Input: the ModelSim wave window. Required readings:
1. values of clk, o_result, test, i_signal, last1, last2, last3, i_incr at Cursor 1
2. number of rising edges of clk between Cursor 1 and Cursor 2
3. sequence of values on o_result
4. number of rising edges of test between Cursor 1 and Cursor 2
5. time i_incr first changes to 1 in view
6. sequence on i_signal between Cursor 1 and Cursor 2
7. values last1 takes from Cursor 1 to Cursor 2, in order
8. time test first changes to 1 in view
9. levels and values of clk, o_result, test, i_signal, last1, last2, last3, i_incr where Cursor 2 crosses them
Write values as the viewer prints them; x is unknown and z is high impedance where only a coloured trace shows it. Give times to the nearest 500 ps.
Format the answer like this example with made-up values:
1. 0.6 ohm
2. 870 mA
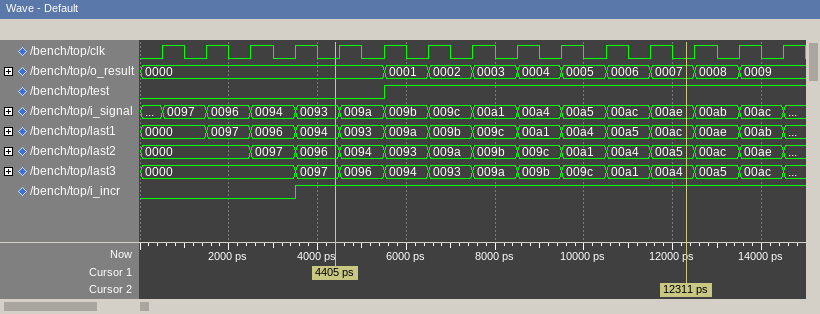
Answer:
1. clk=0, o_result=0000, test=0, i_signal=0093, last1=0094, last2=0096, last3=0097, i_incr=1
2. 8
3. 0000, 0001, 0002, 0003, 0004, 0005, 0006, 0007, 0008, 0009
4. 1
5. 3500 ps
6. 0093, 009a, 009b, 009c, 00a1, 00a4, 00a5, 00ac, 00ae
7. 0094, 0093, 009a, 009b, 009c, 00a1, 00a4, 00a5, 00ac
8. 5500 ps
9. clk=0, o_result=0007, test=1, i_signal=00ae, last1=00ac, last2=00a5, last3=00a4, i_incr=1
